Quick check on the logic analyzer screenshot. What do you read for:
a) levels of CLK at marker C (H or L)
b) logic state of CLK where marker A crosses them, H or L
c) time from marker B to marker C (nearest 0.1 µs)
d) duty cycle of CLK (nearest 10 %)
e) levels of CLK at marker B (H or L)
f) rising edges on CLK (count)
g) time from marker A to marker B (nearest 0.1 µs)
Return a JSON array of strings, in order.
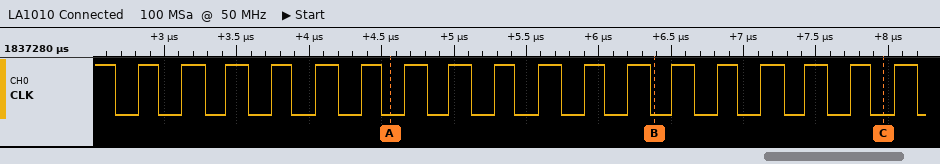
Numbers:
["CLK=L", "CLK=L", "1.6 µs", "50 %", "CLK=L", "18", "1.8 µs"]
